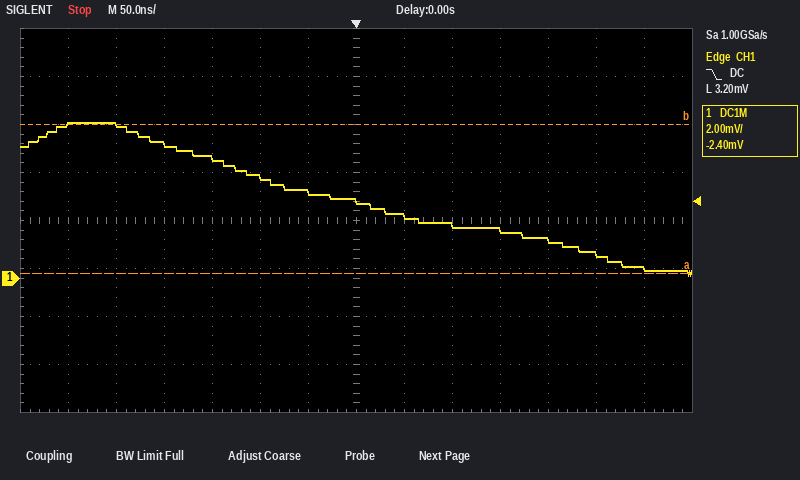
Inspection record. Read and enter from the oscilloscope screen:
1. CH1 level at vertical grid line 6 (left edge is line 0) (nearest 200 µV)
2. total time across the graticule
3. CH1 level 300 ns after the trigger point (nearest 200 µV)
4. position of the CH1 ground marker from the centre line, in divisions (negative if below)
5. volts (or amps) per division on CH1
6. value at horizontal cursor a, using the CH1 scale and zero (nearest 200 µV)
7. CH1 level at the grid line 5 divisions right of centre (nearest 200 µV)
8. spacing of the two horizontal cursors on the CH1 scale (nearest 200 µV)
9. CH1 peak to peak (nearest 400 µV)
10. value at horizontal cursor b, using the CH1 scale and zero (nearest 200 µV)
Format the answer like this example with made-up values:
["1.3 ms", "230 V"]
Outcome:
["3.6 mV", "700 ns", "400 µV", "-1.2 div", "2 mV", "200 µV", "1.0 mV", "6.2 mV", "6.4 mV", "6.4 mV"]
